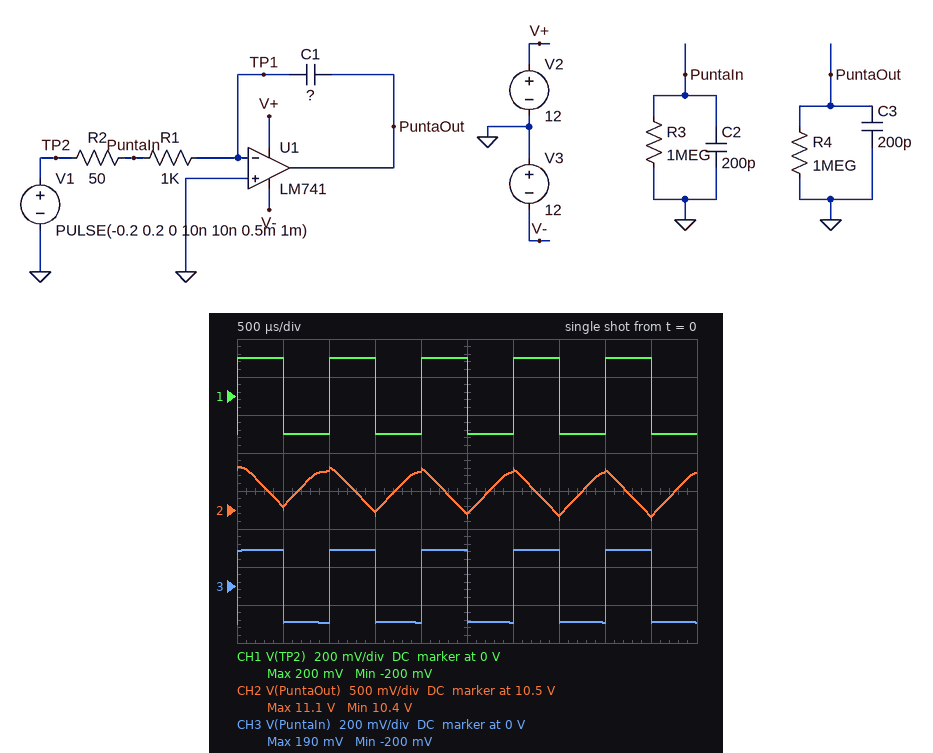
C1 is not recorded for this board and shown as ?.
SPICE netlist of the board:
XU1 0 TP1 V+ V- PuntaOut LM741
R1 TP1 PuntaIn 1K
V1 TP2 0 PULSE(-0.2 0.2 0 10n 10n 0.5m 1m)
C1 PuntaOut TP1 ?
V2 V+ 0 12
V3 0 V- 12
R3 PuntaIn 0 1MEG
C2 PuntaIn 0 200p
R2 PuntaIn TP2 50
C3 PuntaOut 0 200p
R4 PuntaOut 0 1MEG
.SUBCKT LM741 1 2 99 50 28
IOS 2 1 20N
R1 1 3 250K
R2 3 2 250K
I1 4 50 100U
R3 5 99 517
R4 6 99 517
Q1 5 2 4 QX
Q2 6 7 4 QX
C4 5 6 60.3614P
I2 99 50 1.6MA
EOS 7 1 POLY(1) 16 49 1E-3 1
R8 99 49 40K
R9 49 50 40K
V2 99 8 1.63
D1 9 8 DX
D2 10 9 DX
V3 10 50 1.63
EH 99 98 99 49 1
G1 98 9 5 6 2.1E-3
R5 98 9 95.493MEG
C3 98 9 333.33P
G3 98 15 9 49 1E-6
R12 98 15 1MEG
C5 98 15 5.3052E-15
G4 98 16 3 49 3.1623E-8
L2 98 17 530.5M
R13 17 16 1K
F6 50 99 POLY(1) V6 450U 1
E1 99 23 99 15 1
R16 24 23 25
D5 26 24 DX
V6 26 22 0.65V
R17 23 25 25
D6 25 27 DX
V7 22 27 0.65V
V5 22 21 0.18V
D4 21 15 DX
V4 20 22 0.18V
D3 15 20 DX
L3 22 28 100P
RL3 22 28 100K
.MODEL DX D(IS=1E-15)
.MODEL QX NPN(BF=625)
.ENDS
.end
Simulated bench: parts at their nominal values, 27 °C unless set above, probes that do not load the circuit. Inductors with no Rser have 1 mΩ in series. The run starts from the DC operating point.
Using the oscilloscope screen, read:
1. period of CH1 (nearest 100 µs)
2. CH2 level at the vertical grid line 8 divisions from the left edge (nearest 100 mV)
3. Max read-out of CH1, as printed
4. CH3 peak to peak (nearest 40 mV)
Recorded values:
1.0 ms
11.0 V
200 mV
400 mV
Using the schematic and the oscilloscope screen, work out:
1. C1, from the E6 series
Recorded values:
150 nF
